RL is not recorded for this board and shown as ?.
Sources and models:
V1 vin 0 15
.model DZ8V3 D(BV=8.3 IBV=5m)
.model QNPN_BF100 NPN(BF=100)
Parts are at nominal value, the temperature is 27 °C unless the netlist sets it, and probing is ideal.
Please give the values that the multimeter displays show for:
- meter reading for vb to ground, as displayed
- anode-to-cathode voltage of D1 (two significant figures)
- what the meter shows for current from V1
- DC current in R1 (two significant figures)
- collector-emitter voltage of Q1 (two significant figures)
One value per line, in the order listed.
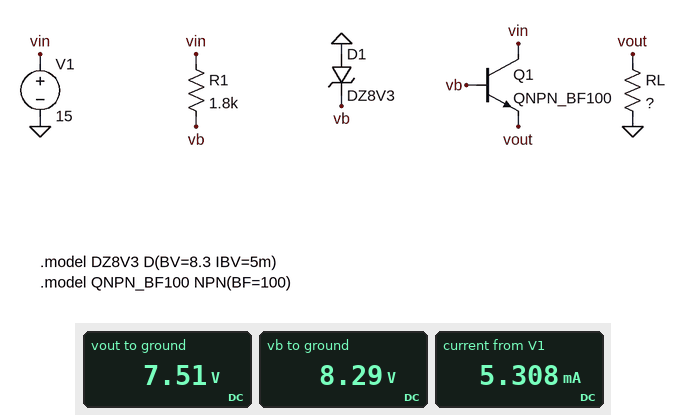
8.29 V
-8.3 V
5.308 mA
3.7 mA
7.5 V
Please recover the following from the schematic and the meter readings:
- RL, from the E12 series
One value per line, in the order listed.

4.7 kΩ
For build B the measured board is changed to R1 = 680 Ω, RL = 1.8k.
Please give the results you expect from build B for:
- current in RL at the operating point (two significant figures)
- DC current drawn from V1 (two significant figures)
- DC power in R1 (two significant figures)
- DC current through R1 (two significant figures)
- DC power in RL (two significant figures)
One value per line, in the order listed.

4.2 mA
14 mA
66 mW
9.8 mA
31 mW
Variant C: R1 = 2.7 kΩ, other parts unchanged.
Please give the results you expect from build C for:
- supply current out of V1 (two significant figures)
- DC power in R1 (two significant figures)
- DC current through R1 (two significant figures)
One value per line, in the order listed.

4.1 mA
17 mW
2.5 mA
